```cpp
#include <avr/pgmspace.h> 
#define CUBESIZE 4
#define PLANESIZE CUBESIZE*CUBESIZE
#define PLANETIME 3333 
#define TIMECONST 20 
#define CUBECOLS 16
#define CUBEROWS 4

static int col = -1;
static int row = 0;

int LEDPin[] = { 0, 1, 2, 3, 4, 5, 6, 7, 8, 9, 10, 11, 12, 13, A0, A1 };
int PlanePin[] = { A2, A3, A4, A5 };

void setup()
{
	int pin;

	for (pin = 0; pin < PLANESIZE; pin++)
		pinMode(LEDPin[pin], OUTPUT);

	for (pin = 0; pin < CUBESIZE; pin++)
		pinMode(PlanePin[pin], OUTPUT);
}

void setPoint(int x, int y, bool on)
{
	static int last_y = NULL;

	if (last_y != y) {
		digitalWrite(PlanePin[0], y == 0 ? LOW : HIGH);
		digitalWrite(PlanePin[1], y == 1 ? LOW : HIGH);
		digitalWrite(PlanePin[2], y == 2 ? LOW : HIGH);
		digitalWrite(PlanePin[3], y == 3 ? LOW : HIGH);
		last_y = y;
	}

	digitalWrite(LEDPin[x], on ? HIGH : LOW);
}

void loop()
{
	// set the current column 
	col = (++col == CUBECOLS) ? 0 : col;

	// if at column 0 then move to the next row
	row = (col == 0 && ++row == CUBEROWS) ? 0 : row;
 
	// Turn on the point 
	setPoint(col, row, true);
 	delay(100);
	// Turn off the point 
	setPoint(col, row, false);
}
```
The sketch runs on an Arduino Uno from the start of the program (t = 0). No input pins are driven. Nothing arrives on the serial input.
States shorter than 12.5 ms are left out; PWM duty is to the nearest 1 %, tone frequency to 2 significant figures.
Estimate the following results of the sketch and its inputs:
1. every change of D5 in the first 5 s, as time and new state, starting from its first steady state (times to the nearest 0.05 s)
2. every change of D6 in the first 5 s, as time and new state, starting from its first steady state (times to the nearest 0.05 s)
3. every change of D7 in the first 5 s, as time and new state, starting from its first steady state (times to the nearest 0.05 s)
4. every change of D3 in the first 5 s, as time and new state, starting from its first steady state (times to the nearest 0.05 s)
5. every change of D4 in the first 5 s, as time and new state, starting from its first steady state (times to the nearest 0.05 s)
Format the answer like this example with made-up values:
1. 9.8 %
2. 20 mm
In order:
1. 0 s low; 0.5 s high; 0.6 s low; 2.1 s high; 2.2 s low; 3.7 s high; 3.8 s low
2. 0 s low; 0.6 s high; 0.7 s low; 2.2 s high; 2.3 s low; 3.8 s high; 3.9 s low
3. 0 s low; 0.7 s high; 0.8 s low; 2.3 s high; 2.4 s low; 3.9 s high; 4 s low
4. 0 s low; 0.3 s high; 0.4 s low; 1.9 s high; 2 s low; 3.5 s high; 3.6 s low
5. 0 s low; 0.4 s high; 0.5 s low; 2 s high; 2.1 s low; 3.6 s high; 3.7 s low
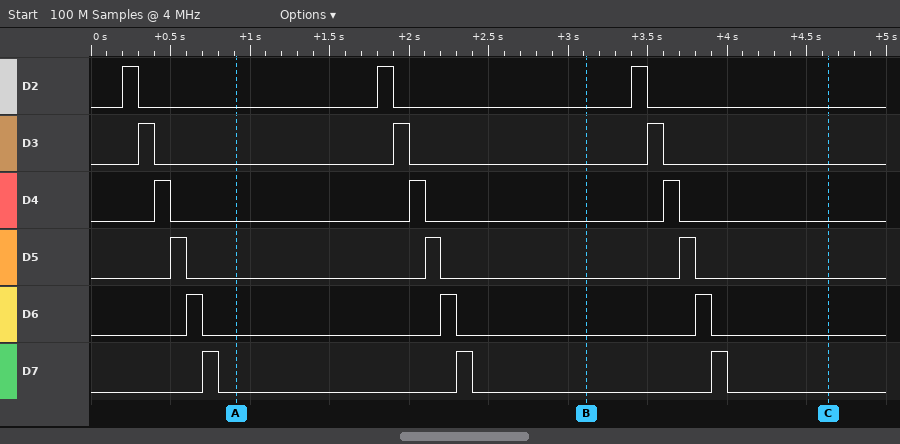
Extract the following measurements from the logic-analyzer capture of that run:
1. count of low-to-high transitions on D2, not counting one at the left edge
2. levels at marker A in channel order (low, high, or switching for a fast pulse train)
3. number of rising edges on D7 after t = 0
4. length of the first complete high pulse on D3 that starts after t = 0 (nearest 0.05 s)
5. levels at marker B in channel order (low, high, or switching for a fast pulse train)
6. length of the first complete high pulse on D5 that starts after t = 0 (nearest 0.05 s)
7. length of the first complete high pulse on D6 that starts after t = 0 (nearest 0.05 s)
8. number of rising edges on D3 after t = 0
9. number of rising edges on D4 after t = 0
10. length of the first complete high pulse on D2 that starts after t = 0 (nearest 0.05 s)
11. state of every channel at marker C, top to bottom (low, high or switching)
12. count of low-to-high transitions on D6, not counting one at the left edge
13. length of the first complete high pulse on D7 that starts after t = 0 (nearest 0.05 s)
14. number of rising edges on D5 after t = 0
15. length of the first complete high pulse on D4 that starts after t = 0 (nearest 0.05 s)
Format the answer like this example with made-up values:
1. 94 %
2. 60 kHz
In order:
1. 3
2. D2 low, D3 low, D4 low, D5 low, D6 low, D7 low
3. 3
4. 0.10 s
5. D2 low, D3 low, D4 low, D5 low, D6 low, D7 low
6. 0.10 s
7. 0.10 s
8. 3
9. 3
10. 0.10 s
11. D2 low, D3 low, D4 low, D5 low, D6 low, D7 low
12. 3
13. 0.10 s
14. 3
15. 0.10 s
